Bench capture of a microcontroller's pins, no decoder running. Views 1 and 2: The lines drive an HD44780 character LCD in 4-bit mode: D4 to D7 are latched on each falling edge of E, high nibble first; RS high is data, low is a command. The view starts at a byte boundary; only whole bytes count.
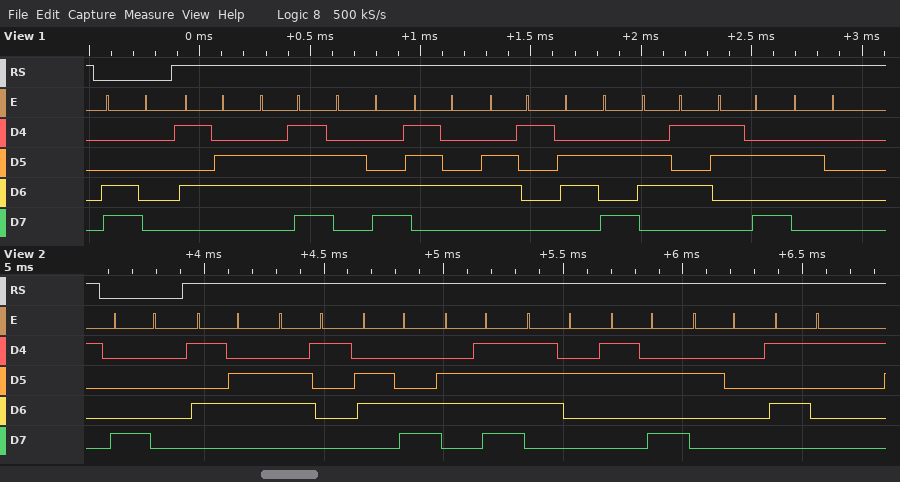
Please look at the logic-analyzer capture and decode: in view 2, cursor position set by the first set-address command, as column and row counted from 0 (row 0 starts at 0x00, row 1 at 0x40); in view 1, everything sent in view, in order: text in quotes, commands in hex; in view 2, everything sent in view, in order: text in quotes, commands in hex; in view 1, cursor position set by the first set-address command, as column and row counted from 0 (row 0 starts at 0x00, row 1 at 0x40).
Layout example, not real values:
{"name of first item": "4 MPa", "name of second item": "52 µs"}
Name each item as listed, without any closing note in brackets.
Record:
{"in view 2, cursor position set by the first set-address command, as column and row counted from 0": "column 0, row 0", "in view 1, everything sent in view, in order: text in quotes, commands in hex": "0xC0 \"Voltaje: \"", "in view 2, everything sent in view, in order: text in quotes, commands in hex": "0x80 \"Valor: Q\"", "in view 1, cursor position set by the first set-address command, as column and row counted from 0": "column 0, row 1"}
